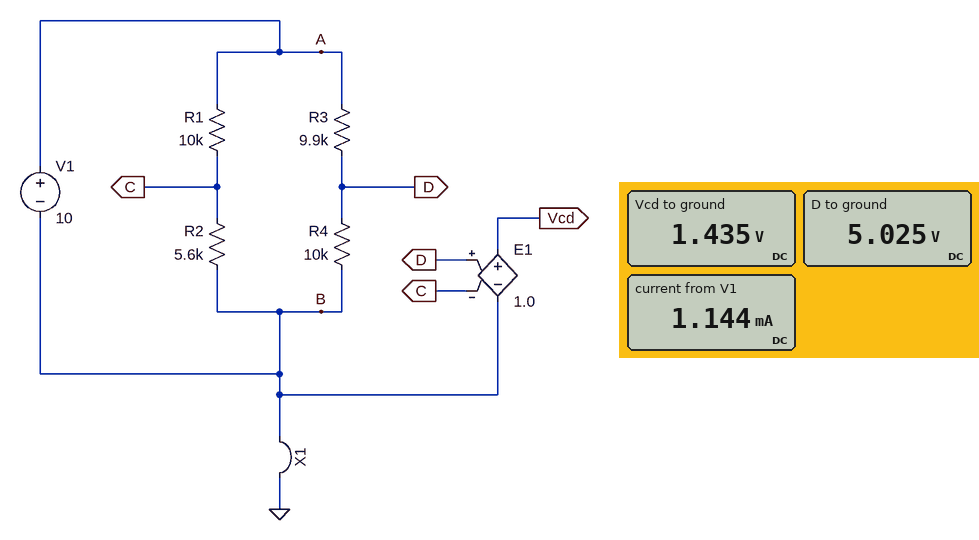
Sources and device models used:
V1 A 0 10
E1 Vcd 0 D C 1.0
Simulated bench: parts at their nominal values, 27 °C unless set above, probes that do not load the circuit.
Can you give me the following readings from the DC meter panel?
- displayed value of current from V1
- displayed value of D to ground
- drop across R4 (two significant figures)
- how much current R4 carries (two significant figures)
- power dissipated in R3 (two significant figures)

1.144 mA
5.025 V
5.0 V
500 µA
2.5 mW
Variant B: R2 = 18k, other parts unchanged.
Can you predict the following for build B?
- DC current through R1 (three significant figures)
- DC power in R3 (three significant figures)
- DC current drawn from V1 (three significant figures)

357 µA
2.50 mW
860 µA
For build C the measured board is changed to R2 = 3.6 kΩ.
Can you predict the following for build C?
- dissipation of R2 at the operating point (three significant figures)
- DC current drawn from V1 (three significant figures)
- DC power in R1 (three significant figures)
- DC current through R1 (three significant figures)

1.95 mW
1.24 mA
5.41 mW
735 µA
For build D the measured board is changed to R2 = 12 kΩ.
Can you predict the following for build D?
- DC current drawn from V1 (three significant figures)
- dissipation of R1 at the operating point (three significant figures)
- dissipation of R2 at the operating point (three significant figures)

957 µA
2.07 mW
2.48 mW
